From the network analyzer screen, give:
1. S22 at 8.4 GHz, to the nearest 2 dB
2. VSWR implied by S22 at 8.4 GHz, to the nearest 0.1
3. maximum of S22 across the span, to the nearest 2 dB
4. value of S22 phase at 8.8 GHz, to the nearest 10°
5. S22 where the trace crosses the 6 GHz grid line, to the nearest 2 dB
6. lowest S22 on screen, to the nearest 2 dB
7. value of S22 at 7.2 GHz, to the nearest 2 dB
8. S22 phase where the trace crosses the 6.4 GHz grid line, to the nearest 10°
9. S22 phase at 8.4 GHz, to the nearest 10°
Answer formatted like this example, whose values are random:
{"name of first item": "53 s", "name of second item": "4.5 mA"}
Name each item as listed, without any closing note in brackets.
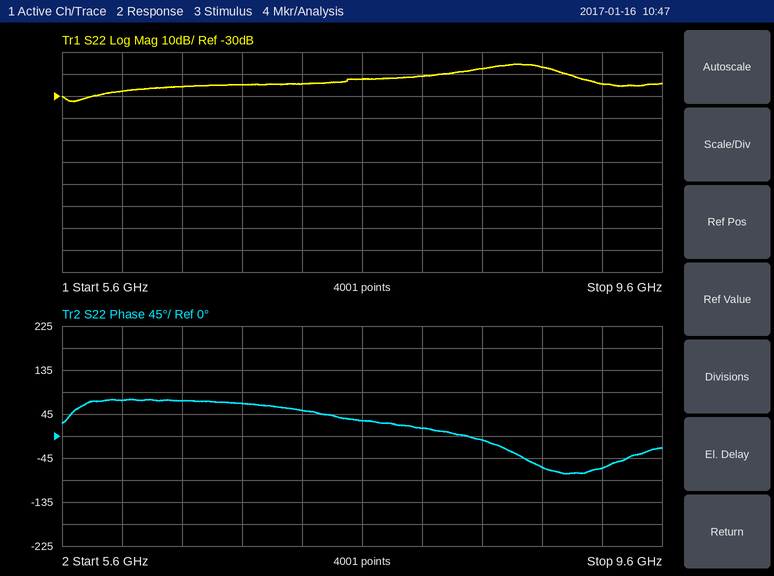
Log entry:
{"S22 at 8.4 GHz, to the nearest 2 dB": "-18 dB", "VSWR implied by S22 at 8.4 GHz, to the nearest 0.1": "1.3", "maximum of S22 across the span, to the nearest 2 dB": "-16 dB", "value of S22 phase at 8.8 GHz, to the nearest 10°": "-60°", "S22 where the trace crosses the 6 GHz grid line, to the nearest 2 dB": "-28 dB", "lowest S22 on screen, to the nearest 2 dB": "-32 dB", "value of S22 at 7.2 GHz, to the nearest 2 dB": "-24 dB", "S22 phase where the trace crosses the 6.4 GHz grid line, to the nearest 10°": "70°", "S22 phase at 8.4 GHz, to the nearest 10°": "-10°"}
